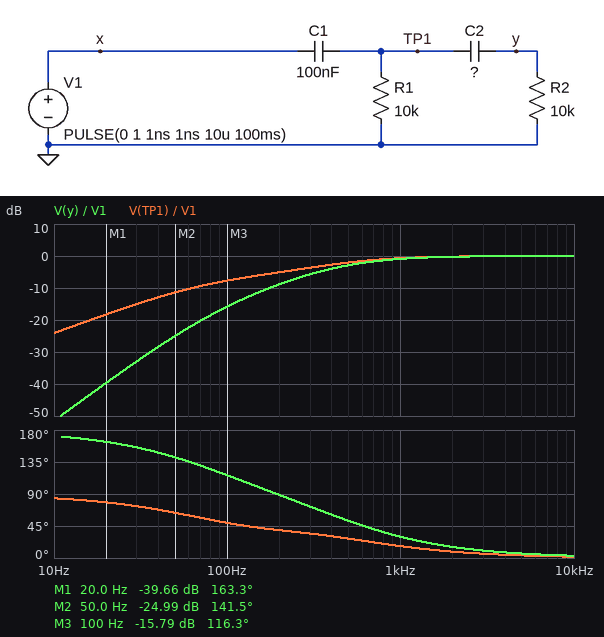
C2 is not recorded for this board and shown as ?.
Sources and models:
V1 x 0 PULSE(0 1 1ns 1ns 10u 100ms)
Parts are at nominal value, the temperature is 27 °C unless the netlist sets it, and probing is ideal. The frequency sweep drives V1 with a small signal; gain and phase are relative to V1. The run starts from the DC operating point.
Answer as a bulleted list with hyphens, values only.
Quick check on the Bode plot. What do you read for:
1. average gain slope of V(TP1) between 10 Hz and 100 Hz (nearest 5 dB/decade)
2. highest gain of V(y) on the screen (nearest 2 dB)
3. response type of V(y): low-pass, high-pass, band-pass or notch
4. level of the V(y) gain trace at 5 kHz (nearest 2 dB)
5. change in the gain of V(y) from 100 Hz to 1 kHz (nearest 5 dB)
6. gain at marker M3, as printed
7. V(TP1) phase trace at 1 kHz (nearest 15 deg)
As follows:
- 15 dB/decade
- 0 dB
- high-pass
- 0 dB
- 15 dB
- -15.79 dB
- 15 deg
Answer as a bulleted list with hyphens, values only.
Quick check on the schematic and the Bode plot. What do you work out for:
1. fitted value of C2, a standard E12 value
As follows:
- 68 nF
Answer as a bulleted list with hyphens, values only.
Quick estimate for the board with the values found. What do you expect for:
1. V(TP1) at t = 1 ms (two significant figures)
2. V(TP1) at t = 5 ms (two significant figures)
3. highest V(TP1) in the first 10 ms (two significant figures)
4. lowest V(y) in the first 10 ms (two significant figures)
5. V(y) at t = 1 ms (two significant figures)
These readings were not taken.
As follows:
- 270 mV
- 33 mV
- 1.0 V
- -81 mV
- -60 mV
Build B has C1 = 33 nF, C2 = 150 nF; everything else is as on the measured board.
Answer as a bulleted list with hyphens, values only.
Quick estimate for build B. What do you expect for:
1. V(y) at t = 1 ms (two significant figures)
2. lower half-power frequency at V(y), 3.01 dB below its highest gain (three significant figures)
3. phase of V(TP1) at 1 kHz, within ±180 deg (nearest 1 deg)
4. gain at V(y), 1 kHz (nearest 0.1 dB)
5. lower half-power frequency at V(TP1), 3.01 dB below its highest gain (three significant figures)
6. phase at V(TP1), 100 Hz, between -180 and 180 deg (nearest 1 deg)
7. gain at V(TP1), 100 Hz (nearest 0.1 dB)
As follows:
- -36 mV
- 1.02 kHz
- 42 deg
- -3.1 dB
- 1.01 kHz
- 64 deg
- -17.9 dB
